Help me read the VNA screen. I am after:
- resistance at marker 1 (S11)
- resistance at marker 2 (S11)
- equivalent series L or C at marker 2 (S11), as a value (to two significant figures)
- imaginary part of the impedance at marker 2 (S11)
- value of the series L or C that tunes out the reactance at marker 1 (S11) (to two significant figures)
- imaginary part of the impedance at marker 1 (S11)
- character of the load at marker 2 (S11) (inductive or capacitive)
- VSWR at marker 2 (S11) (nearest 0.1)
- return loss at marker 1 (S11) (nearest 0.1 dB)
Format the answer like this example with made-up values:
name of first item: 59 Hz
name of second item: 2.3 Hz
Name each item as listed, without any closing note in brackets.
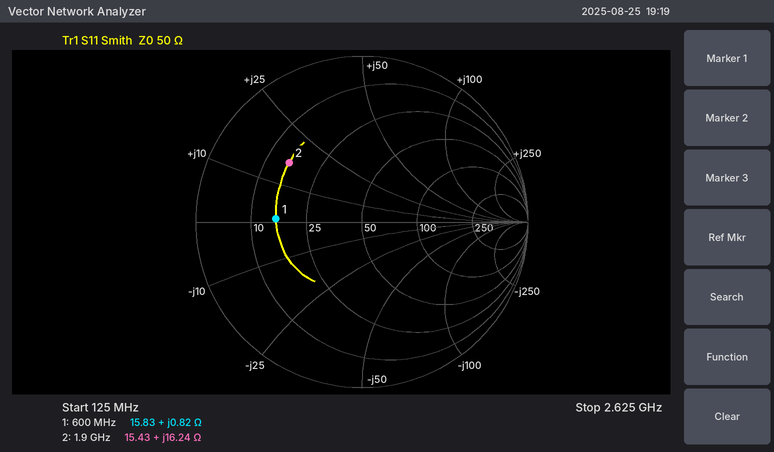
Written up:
resistance at marker 1: 15.83 Ω
resistance at marker 2: 15.43 Ω
equivalent series L or C at marker 2 (S11), as a value: 1.4 nH
imaginary part of the impedance at marker 2: +16.24 Ω
value of the series L or C that tunes out the reactance at marker 1 (S11): 320 pF
imaginary part of the impedance at marker 1: +0.82 Ω
character of the load at marker 2 (S11): inductive
VSWR at marker 2 (S11): 3.6
return loss at marker 1 (S11): 5.7 dB
